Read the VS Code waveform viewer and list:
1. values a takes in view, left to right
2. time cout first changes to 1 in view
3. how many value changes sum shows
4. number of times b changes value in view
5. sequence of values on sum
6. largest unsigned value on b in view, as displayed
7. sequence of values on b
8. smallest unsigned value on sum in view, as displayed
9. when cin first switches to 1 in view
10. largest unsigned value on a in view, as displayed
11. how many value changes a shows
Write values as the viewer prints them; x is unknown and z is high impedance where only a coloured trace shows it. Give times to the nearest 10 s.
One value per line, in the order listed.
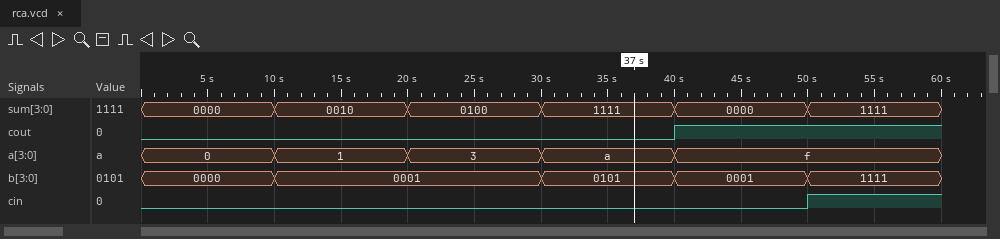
0, 1, 3, a, f
40 s
5
4
0000, 0010, 0100, 1111, 0000, 1111
1111
0000, 0001, 0101, 0001, 1111
0000
50 s
f
4
